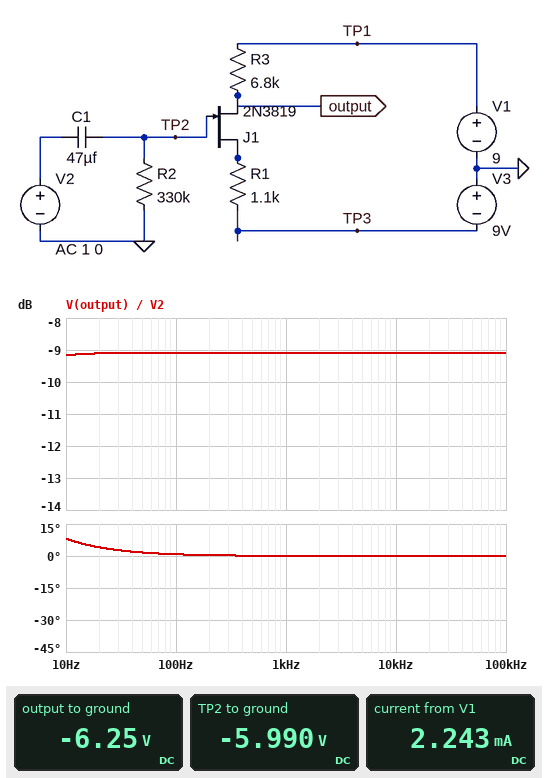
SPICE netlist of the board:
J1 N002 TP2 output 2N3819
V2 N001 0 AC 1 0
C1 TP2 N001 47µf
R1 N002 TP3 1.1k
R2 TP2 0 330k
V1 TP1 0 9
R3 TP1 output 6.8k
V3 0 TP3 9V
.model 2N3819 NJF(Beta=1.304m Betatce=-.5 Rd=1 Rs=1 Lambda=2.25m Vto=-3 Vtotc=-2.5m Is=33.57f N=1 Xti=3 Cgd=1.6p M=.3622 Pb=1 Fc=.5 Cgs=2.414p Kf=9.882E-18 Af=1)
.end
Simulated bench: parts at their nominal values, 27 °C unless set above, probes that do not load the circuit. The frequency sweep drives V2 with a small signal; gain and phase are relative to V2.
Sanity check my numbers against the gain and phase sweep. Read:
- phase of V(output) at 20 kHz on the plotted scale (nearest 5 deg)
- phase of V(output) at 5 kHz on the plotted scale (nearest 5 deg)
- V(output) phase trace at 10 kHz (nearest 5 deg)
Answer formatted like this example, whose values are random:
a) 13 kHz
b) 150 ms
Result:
a) 0 deg
b) 0 deg
c) 0 deg
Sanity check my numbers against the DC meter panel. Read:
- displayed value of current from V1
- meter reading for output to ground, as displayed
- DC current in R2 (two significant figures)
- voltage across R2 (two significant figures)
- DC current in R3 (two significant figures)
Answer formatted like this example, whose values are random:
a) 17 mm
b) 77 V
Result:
a) 2.243 mA
b) -6.25 V
c) 18 µA
d) 6.0 V
e) 2.2 mA
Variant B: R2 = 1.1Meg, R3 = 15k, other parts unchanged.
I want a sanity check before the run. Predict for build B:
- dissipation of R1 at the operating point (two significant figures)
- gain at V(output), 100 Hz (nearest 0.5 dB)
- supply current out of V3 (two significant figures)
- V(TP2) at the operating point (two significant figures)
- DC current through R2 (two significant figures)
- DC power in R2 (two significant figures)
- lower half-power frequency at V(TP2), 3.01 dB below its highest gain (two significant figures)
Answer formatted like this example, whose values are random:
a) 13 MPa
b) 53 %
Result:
a) 1.4 mW
b) -15.0 dB
c) 1.1 mA
d) -7.3 V
e) 6.6 µA
f) 48 µW
g) 690 mHz
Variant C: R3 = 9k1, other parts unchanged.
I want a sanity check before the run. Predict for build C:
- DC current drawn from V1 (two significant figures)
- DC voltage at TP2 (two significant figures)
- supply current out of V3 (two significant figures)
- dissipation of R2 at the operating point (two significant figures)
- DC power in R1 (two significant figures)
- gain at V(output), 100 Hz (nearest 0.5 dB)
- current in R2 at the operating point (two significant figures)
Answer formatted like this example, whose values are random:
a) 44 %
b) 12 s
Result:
a) 1.7 mA
b) -6.5 V
c) 1.8 mA
d) 130 µW
e) 3.4 mW
f) -8.0 dB
g) 20 µA
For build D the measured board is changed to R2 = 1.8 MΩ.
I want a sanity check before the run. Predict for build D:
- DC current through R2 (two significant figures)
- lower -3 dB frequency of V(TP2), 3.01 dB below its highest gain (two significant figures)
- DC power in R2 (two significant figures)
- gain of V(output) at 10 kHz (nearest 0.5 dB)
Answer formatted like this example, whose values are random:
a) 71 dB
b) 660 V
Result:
a) 3.4 µA
b) 390 mHz
c) 20 µW
d) -26.5 dB
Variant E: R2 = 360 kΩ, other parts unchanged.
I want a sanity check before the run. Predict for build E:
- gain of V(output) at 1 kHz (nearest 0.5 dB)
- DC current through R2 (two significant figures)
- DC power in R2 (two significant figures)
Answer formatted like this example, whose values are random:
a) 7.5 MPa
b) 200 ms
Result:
a) -9.5 dB
b) 17 µA
c) 100 µW
